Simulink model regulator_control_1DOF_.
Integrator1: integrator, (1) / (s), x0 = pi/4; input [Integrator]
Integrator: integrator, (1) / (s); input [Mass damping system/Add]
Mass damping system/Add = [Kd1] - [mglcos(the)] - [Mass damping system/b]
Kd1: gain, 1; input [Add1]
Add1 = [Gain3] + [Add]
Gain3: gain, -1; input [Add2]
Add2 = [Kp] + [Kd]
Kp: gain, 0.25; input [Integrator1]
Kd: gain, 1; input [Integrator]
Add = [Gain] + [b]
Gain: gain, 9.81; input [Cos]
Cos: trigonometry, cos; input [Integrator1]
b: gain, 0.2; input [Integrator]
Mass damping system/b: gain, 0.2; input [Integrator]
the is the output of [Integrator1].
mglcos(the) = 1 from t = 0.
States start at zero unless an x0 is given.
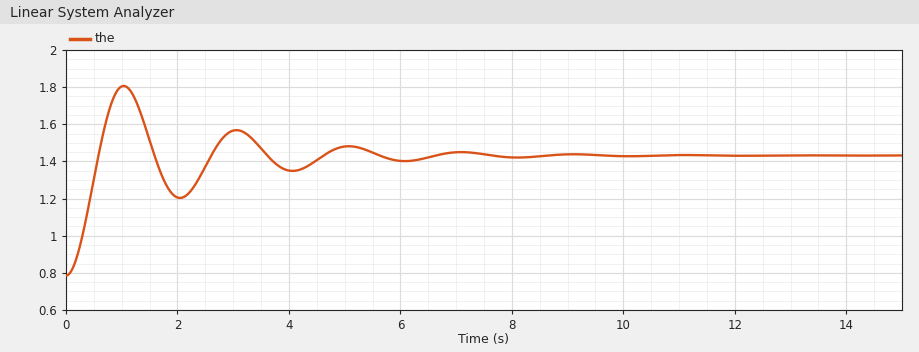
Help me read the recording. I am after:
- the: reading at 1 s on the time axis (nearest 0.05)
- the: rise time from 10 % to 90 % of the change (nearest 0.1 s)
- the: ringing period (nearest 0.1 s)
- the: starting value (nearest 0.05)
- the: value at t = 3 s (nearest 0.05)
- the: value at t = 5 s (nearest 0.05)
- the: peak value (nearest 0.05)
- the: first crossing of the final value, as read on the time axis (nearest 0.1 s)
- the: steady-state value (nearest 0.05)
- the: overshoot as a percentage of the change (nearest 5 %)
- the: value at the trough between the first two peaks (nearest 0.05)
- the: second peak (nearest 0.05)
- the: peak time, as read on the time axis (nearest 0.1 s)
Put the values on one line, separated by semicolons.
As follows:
1.80; 0.4 s; 2.0 s; 0.80; 1.55; 1.50; 1.80; 0.6 s; 1.45; 60 %; 1.20; 1.55; 1.0 s
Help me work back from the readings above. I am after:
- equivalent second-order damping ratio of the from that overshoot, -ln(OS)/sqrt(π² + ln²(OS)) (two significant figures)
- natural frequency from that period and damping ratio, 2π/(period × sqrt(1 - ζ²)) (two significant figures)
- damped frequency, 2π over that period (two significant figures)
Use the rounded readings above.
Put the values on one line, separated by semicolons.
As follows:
0.16; 3.2 rad/s; 3.1 rad/s
